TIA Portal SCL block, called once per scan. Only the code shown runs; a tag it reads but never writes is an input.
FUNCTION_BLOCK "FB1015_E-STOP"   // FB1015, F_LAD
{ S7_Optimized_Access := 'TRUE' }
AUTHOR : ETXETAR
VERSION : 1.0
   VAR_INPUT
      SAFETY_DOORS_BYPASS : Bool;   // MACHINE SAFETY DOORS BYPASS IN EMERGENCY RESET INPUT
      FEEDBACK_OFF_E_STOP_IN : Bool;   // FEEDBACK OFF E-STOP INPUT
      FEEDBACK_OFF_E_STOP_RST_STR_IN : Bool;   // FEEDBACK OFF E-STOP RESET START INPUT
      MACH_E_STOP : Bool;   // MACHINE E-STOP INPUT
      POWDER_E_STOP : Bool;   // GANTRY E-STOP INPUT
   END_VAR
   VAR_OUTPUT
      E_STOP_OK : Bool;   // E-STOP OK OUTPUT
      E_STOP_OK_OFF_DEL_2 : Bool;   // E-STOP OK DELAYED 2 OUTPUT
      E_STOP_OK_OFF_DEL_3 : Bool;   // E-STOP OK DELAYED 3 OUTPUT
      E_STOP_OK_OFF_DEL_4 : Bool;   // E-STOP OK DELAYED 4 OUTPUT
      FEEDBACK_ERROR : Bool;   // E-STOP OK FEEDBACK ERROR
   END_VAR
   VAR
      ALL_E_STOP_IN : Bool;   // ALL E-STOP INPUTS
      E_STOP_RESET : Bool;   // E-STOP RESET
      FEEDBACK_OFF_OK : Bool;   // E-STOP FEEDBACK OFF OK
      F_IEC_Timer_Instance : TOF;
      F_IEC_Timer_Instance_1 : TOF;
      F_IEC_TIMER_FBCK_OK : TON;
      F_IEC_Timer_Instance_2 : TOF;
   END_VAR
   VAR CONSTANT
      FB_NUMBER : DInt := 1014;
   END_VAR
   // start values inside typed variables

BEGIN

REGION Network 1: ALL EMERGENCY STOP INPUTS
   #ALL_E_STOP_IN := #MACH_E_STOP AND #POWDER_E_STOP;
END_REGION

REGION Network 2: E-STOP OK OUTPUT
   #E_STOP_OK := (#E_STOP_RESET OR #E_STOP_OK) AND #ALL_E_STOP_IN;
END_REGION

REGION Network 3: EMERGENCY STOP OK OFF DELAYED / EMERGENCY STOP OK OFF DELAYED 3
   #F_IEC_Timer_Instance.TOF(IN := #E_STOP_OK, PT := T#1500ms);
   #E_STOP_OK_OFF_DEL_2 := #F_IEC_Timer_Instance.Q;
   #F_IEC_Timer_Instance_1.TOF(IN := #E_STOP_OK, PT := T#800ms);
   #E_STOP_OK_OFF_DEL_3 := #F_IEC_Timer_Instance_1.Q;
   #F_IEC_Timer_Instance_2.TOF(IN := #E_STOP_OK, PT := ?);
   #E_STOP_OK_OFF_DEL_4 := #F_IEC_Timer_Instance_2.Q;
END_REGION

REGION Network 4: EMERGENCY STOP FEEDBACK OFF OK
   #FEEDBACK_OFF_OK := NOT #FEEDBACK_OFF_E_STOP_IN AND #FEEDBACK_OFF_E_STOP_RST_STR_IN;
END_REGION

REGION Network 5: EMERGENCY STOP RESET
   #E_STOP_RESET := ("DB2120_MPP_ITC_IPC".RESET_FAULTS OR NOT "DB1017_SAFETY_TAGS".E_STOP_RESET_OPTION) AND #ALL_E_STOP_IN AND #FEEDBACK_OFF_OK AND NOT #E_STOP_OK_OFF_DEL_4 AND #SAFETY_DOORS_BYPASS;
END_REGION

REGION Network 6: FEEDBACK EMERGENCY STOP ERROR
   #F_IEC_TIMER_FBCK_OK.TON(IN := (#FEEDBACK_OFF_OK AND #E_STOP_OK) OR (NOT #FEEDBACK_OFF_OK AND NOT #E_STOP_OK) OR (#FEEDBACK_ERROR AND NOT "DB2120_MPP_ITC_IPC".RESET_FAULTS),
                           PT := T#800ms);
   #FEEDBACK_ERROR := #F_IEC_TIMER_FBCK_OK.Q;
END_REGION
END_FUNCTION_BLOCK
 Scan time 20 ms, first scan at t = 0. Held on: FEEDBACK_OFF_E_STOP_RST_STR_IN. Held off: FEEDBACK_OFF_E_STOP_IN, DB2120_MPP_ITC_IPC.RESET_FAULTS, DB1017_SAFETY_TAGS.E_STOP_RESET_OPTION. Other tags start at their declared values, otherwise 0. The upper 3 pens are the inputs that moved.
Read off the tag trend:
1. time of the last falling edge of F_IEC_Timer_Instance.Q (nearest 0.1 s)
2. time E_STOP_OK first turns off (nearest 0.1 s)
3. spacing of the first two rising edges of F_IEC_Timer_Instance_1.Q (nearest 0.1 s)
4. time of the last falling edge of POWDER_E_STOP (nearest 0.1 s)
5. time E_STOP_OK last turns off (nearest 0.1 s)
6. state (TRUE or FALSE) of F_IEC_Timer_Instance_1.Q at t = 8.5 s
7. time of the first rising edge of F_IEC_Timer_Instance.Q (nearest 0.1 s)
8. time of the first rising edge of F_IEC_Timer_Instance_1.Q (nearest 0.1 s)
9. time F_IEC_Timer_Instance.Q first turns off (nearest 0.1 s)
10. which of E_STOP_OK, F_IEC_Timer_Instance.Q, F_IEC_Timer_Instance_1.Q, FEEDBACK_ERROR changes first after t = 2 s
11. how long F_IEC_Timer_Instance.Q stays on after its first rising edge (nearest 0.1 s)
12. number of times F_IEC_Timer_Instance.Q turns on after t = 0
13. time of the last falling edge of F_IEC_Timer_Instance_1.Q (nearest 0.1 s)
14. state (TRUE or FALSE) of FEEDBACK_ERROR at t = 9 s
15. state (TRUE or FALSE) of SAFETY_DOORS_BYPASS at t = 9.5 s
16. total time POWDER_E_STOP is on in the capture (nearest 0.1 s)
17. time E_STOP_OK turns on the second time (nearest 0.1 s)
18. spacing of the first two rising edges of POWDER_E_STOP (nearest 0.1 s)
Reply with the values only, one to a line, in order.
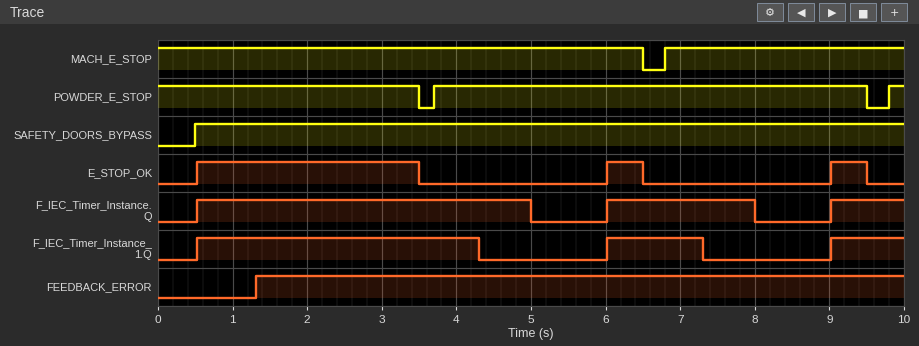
8.0 s
3.5 s
5.5 s
9.5 s
9.5 s
FALSE
0.5 s
0.5 s
5.0 s
E_STOP_OK
4.5 s
3
7.3 s
TRUE
TRUE
9.5 s
6.0 s
6.1 s
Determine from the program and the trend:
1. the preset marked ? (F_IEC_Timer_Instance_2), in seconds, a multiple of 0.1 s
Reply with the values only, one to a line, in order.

2.5 s
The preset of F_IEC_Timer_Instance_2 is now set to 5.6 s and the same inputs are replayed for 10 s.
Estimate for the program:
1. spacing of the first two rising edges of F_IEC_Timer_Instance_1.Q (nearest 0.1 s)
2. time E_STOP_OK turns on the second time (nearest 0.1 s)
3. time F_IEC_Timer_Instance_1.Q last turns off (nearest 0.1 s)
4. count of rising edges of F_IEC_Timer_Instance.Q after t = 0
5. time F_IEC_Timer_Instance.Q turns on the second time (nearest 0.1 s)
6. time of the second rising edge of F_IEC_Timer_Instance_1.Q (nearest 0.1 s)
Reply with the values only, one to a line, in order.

8.6 s
9.1 s
4.3 s
2
9.1 s
9.1 s
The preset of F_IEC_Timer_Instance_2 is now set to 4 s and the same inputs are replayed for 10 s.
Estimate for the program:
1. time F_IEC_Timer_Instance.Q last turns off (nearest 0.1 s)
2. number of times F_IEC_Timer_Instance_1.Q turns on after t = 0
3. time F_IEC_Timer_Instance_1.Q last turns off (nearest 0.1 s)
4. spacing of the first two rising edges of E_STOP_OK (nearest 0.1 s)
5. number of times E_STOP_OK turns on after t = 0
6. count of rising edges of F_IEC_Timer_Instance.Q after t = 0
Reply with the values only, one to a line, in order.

5.0 s
2
4.3 s
7.0 s
2
2
